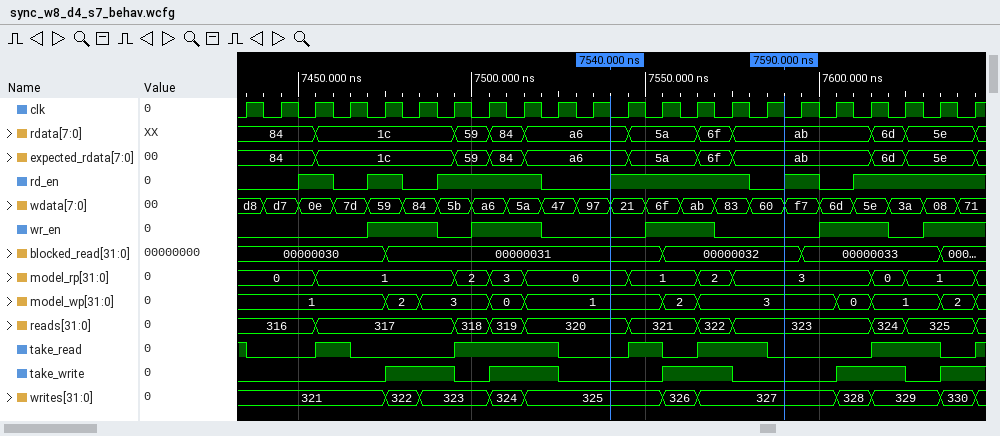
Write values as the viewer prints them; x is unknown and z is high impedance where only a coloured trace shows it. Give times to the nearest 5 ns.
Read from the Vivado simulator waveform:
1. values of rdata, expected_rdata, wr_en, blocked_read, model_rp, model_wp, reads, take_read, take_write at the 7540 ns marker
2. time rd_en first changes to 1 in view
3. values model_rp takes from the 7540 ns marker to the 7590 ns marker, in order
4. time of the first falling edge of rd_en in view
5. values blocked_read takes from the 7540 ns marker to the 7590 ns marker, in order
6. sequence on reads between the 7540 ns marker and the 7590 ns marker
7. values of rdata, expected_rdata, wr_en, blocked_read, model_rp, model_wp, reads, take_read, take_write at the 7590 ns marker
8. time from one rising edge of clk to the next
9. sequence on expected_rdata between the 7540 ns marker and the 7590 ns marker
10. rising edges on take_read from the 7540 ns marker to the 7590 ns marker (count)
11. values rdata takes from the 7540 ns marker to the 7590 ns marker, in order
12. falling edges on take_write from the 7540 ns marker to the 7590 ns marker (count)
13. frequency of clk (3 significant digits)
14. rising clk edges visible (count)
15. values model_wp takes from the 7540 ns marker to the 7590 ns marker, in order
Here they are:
rdata=a6, expected_rdata=a6, wr_en=0, blocked_read=00000031, model_rp=0, model_wp=1, reads=320, take_read=0, take_write=0
7450 ns
0, 1, 2, 3
7460 ns
00000031, 00000032
320, 321, 322, 323
rdata=ab, expected_rdata=ab, wr_en=0, blocked_read=00000032, model_rp=3, model_wp=3, reads=323, take_read=0, take_write=0
10 ns
a6, 5a, 6f, ab
2
a6, 5a, 6f, ab
1
100 MHz
22
1, 2, 3
